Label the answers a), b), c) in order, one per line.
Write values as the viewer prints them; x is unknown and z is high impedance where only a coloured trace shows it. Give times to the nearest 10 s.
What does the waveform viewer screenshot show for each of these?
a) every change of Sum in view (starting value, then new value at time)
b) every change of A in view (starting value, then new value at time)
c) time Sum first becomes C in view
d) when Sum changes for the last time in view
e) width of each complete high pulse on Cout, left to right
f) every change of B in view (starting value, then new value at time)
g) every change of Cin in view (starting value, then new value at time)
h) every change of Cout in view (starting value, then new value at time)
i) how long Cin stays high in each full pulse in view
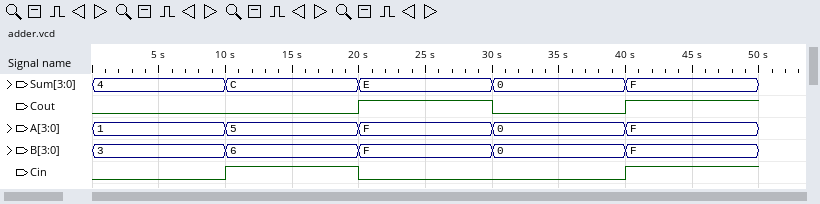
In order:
a) 4, C at 10 s, E at 20 s, 0 at 30 s, F at 40 s
b) 1, 5 at 10 s, F at 20 s, 0 at 30 s, F at 40 s
c) 10 s
d) 40 s
e) 10 s
f) 3, 6 at 10 s, F at 20 s, 0 at 30 s, F at 40 s
g) 0, 1 at 10 s, 0 at 20 s, 1 at 40 s
h) 0, 1 at 20 s, 0 at 30 s, 1 at 40 s
i) 10 s
